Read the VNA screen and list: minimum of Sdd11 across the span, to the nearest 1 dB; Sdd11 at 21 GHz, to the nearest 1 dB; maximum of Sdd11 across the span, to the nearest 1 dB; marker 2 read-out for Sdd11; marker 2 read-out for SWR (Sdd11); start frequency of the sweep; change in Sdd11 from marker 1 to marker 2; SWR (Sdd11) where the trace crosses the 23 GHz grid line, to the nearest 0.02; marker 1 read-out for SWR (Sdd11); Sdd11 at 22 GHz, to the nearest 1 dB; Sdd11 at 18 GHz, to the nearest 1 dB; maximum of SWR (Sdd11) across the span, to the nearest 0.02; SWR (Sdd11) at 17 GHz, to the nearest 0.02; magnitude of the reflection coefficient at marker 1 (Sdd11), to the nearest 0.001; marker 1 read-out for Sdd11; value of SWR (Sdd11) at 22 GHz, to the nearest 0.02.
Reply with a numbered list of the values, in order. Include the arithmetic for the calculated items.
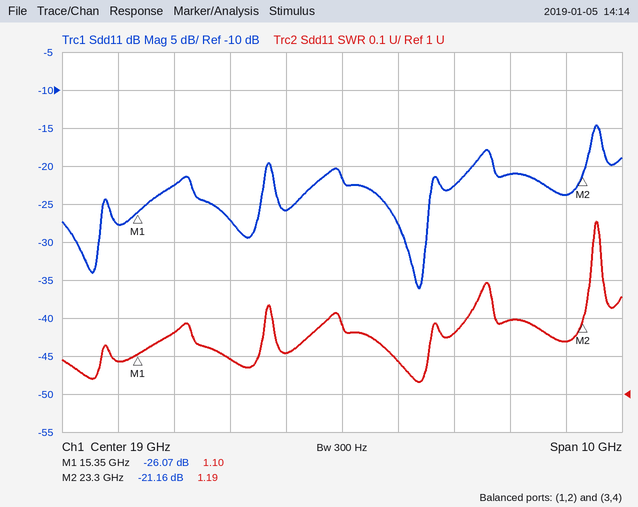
1. -36 dB
2. -23 dB
3. -15 dB
4. -21.16 dB
5. 1.19
6. 14 GHz
7. -21.16 − (-26.07) = 4.91 dB
8. 1.14
9. 1.10
10. -21 dB
11. -26 dB
12. 1.46
13. 1.10
14. 10^(-26.07/20) ≈ 0.050
15. -26.07 dB
16. 1.20
